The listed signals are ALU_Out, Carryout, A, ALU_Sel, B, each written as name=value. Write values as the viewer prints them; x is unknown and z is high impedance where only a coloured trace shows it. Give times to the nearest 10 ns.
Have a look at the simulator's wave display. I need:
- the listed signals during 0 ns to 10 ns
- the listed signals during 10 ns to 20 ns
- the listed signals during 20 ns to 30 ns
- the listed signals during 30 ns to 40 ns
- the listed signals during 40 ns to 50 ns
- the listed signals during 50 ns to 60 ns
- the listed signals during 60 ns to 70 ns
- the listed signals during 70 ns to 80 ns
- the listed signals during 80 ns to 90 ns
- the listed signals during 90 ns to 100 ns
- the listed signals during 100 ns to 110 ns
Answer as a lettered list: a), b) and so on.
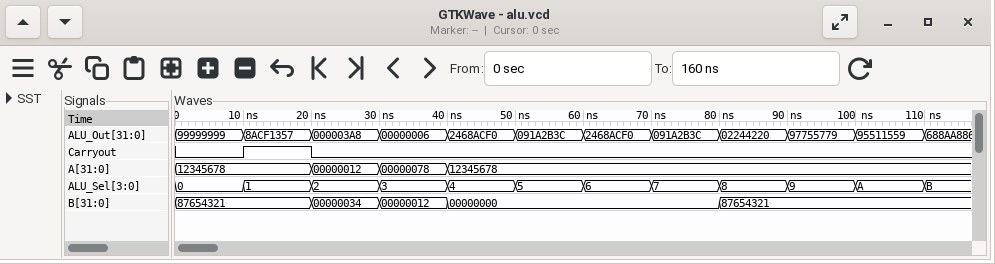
a) ALU_Out=99999999, Carryout=0, A=12345678, ALU_Sel=0, B=87654321
b) ALU_Out=8ACF1357, Carryout=1, A=12345678, ALU_Sel=1, B=87654321
c) ALU_Out=000003A8, Carryout=0, A=00000012, ALU_Sel=2, B=00000034
d) ALU_Out=00000006, Carryout=0, A=00000078, ALU_Sel=3, B=00000012
e) ALU_Out=2468ACF0, Carryout=0, A=12345678, ALU_Sel=4, B=00000000
f) ALU_Out=091A2B3C, Carryout=0, A=12345678, ALU_Sel=5, B=00000000
g) ALU_Out=2468ACF0, Carryout=0, A=12345678, ALU_Sel=6, B=00000000
h) ALU_Out=091A2B3C, Carryout=0, A=12345678, ALU_Sel=7, B=00000000
i) ALU_Out=02244220, Carryout=0, A=12345678, ALU_Sel=8, B=87654321
j) ALU_Out=97755779, Carryout=0, A=12345678, ALU_Sel=9, B=87654321
k) ALU_Out=95511559, Carryout=0, A=12345678, ALU_Sel=A, B=87654321
